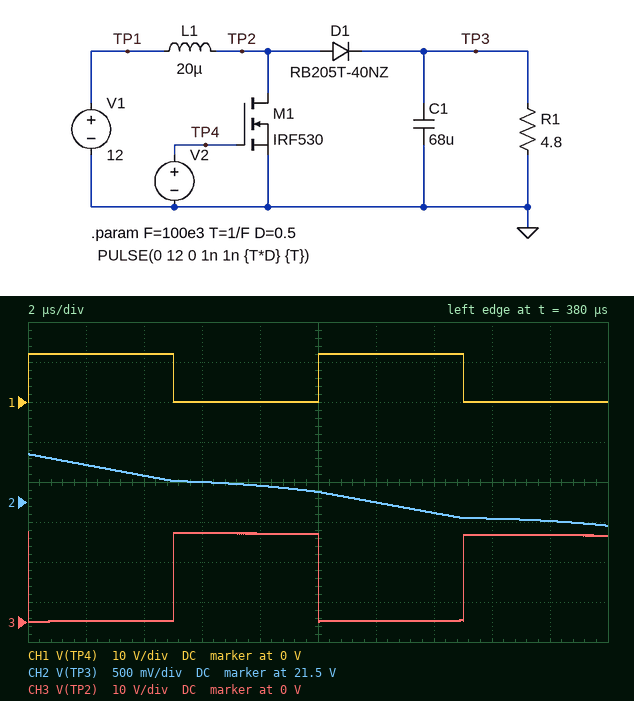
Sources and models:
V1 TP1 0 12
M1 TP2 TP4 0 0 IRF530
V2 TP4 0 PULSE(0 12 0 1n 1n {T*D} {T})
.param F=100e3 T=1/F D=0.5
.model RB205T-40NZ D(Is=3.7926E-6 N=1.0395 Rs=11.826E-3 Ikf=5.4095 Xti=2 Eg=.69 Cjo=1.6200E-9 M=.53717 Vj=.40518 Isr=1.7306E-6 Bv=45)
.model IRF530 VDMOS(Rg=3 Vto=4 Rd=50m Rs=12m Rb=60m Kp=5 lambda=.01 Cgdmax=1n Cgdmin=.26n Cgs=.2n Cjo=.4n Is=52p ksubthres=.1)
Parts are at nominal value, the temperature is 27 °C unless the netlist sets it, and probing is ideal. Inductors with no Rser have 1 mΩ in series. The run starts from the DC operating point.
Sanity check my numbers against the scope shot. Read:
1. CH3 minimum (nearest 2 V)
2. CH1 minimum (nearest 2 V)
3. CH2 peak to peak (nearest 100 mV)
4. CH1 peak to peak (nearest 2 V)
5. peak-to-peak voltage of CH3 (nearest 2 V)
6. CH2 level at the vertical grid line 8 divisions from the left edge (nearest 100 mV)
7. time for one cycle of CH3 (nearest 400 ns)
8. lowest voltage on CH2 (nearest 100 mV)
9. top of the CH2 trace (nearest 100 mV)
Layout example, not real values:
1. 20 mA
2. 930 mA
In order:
1. 0 V
2. 0 V
3. 900 mV
4. 12 V
5. 22 V
6. 21.3 V
7. 10.0 µs
8. 21.2 V
9. 22.1 V
